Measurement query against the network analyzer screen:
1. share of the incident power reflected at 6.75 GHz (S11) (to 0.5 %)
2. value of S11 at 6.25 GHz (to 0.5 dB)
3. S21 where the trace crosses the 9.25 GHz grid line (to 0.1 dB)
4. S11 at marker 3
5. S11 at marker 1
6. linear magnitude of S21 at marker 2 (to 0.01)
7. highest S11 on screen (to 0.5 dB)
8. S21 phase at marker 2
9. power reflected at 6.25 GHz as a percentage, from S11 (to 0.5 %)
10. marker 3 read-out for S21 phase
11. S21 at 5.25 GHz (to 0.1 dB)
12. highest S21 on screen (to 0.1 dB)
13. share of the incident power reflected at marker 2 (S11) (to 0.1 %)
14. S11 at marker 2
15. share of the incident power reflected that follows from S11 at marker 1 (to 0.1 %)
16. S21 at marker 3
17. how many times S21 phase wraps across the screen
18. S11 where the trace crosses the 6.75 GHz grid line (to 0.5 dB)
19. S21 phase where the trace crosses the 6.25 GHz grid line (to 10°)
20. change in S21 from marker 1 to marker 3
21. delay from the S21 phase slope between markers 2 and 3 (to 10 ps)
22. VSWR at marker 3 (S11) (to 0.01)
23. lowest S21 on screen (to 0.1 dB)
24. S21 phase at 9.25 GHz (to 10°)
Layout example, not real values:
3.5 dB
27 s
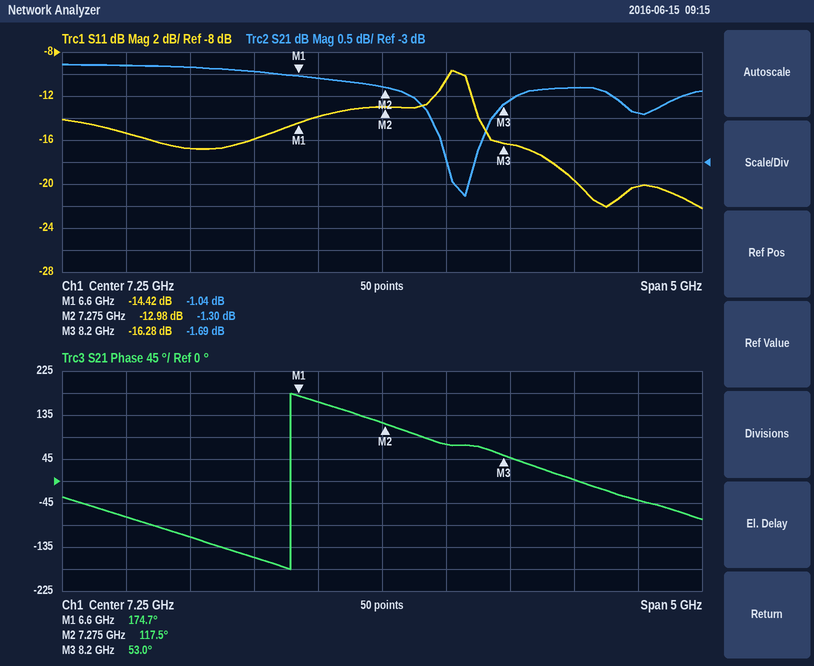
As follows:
4.0 %
-16.0 dB
-1.9 dB
-16.28 dB
-14.42 dB
0.86
-9.5 dB
117.5°
2.5 %
53.0°
-0.8 dB
-0.8 dB
5.0 %
-12.98 dB
3.6 %
-1.69 dB
1
-14.0 dB
-160°
-0.65 dB
190 ps
1.36
-3.8 dB
-40°
